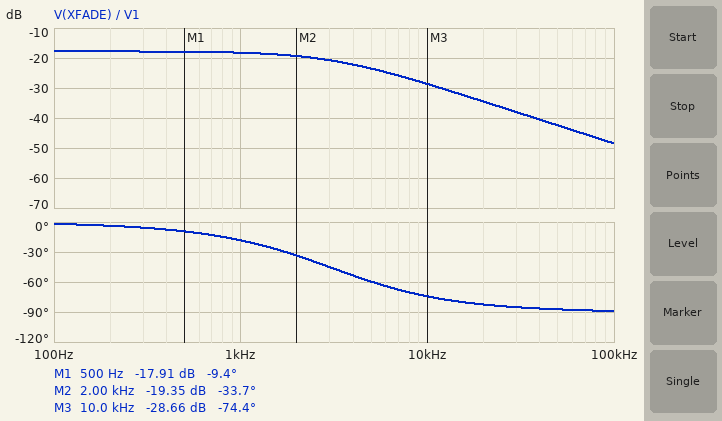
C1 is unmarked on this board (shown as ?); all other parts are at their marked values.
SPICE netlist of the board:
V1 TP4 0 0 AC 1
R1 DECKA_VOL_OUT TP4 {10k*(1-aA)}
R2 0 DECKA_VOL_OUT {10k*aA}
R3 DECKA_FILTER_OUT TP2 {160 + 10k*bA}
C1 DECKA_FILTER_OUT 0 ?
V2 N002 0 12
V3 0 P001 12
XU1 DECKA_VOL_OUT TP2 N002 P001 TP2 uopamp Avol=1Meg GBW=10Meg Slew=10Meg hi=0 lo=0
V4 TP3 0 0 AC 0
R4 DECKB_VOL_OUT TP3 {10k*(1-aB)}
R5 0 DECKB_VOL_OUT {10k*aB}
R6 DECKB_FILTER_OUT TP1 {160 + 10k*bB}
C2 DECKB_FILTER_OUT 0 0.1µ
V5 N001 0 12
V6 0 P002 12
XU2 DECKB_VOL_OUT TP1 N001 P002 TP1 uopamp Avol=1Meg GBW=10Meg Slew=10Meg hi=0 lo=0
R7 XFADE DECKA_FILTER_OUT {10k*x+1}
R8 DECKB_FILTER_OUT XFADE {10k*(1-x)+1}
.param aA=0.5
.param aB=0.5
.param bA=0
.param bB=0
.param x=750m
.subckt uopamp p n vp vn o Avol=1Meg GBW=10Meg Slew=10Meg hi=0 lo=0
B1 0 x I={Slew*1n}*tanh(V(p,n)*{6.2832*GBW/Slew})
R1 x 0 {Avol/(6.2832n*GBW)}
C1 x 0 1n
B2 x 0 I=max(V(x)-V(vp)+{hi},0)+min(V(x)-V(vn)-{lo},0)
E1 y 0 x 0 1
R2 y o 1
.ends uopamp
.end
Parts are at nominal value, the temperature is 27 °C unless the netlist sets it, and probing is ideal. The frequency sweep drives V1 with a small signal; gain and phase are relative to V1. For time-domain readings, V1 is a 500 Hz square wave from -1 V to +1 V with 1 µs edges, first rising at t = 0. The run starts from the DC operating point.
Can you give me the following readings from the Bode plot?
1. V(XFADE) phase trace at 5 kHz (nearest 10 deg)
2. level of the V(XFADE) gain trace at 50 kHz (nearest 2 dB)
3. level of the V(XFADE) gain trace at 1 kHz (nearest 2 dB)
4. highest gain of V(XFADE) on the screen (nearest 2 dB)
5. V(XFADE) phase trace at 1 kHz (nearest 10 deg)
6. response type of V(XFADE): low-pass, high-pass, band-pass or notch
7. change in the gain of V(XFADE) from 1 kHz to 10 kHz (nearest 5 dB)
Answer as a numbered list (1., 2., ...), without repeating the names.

1. -60 deg
2. -42 dB
3. -18 dB
4. -18 dB
5. -20 deg
6. low-pass
7. -10 dB
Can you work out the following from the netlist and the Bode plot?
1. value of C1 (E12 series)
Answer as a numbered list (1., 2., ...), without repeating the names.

1. 330 nF
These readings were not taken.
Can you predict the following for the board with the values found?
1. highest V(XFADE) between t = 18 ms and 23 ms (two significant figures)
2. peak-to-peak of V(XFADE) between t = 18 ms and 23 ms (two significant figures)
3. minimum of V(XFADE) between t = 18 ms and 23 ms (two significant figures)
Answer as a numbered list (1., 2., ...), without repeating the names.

1. 130 mV
2. 260 mV
3. -130 mV
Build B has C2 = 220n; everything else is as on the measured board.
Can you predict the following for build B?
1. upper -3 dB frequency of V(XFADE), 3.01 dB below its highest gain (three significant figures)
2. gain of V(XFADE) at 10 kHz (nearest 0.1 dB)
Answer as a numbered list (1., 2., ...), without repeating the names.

1. 2.98 kHz
2. -28.8 dB
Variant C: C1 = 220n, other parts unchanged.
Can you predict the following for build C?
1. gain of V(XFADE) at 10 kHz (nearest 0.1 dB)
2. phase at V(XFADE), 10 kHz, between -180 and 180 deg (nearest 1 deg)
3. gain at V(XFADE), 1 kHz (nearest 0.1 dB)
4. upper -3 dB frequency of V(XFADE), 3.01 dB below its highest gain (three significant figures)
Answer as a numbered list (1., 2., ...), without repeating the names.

1. -25.6 dB
2. -67 deg
3. -18.0 dB
4. 4.52 kHz
